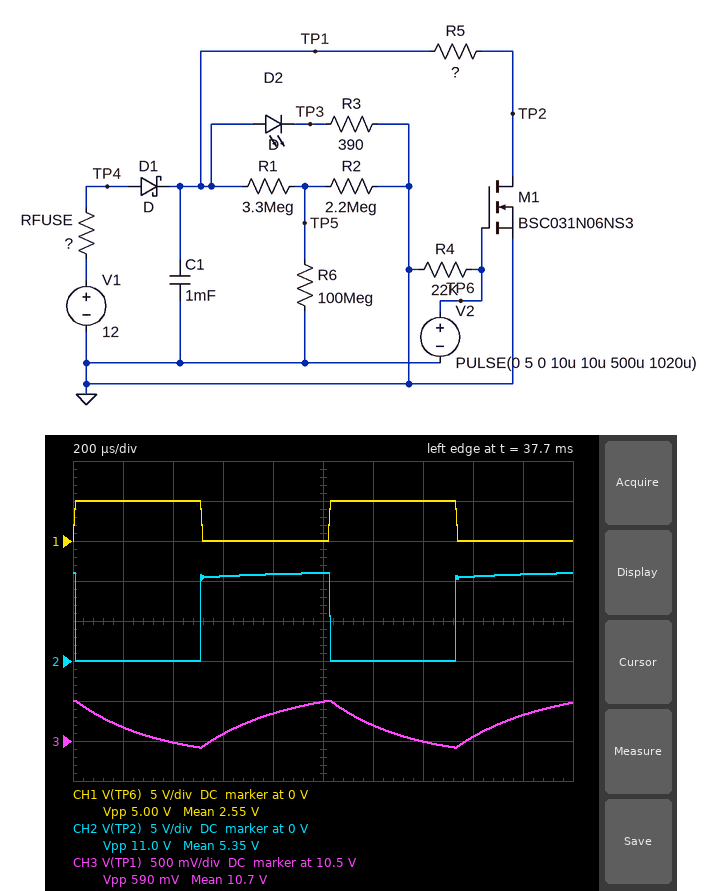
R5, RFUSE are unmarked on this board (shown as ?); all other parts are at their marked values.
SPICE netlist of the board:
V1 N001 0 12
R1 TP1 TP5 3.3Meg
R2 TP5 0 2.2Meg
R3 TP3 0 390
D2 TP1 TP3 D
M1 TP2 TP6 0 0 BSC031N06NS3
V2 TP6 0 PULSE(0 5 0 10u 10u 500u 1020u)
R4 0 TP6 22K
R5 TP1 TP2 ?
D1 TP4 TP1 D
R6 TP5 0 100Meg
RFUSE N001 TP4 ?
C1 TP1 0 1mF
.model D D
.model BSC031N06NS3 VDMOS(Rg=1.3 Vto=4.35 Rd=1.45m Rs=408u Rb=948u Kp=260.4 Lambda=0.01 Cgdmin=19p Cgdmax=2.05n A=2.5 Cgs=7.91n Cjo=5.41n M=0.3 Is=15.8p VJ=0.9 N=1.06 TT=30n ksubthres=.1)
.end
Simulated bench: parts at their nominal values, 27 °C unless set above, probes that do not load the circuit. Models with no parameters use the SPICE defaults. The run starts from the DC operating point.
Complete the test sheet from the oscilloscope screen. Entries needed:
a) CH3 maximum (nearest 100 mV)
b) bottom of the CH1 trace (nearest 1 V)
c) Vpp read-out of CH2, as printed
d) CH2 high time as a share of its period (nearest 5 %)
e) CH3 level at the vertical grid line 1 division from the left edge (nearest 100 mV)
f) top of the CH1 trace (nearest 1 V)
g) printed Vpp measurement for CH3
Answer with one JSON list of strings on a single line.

["11.0 V", "0 V", "11.0 V", "50 %", "10.7 V", "5 V", "590 mV"]
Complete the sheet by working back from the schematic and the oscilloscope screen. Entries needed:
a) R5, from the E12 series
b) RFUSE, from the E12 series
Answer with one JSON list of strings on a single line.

["3.9 Ω", "0.33 Ω"]
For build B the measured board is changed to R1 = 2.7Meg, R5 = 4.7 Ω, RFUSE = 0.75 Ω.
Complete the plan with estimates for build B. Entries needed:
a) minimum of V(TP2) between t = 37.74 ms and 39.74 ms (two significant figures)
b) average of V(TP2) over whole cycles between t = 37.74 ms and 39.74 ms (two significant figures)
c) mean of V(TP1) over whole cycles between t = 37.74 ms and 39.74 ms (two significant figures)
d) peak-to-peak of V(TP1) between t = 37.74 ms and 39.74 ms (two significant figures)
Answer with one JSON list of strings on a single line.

["17 mV", "5.3 V", "10 V", "540 mV"]
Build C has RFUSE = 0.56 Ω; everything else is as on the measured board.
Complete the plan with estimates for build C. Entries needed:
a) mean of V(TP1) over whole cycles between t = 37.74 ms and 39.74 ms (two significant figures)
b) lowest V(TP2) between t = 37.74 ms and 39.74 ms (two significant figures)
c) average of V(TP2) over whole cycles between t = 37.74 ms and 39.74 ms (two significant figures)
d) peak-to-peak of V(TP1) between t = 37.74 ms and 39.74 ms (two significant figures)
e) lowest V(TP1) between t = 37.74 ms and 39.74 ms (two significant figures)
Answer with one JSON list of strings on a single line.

["10 V", "20 mV", "5.3 V", "630 mV", "10 V"]
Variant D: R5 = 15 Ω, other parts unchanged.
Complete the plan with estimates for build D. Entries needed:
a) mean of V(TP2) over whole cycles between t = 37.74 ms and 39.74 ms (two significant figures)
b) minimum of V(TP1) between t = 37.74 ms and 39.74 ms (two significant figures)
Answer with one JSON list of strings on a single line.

["5.6 V", "11 V"]
